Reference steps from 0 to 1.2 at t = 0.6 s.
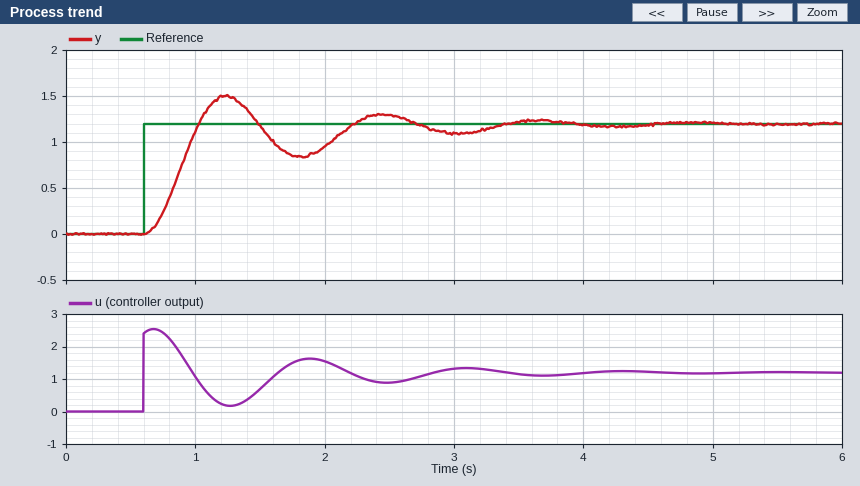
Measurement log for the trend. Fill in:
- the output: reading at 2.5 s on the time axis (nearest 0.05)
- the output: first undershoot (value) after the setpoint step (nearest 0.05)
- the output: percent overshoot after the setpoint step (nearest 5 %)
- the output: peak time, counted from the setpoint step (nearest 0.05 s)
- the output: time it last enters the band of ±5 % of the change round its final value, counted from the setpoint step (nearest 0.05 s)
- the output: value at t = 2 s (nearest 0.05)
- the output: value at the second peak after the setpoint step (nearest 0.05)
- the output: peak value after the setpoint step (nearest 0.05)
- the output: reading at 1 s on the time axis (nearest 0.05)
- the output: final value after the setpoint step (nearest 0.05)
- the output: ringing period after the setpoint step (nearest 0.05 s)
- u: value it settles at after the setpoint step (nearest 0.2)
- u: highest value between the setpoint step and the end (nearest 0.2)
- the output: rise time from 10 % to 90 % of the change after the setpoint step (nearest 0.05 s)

1.30
0.85
25 %
0.65 s
2.65 s
0.95
1.30
1.50
1.10
1.20
1.20 s
1.2
2.6
0.30 s
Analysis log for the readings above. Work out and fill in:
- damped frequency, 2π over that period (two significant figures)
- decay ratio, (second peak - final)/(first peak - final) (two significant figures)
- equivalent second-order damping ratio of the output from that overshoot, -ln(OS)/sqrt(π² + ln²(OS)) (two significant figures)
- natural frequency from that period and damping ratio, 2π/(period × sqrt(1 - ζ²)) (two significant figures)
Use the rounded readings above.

5.2 rad/s
0.33
0.40
5.7 rad/s
